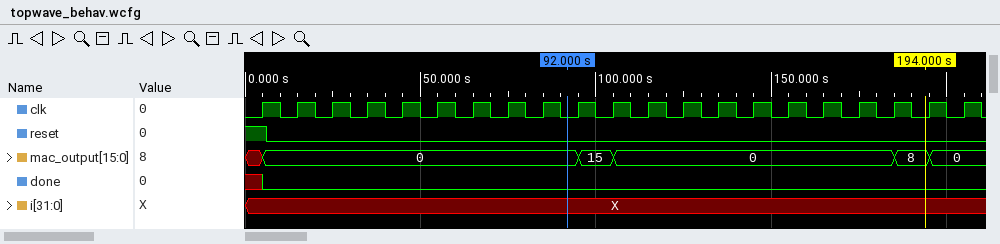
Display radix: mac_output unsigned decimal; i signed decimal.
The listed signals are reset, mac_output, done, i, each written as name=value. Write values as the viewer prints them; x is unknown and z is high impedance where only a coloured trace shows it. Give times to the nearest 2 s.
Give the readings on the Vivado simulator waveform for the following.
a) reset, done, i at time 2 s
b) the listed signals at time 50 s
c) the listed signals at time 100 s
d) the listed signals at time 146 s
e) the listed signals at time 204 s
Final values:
reset=1, done=x, i=X
reset=0, mac_output=0, done=0, i=X
reset=0, mac_output=15, done=0, i=X
reset=0, mac_output=0, done=0, i=X
reset=0, mac_output=0, done=0, i=X
